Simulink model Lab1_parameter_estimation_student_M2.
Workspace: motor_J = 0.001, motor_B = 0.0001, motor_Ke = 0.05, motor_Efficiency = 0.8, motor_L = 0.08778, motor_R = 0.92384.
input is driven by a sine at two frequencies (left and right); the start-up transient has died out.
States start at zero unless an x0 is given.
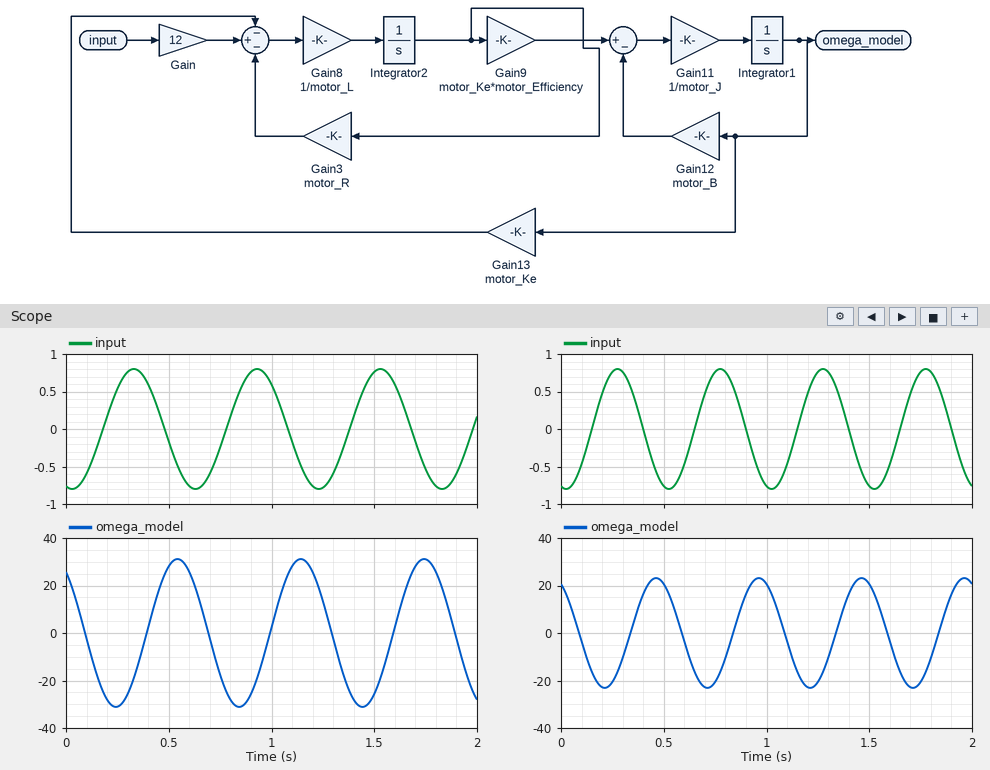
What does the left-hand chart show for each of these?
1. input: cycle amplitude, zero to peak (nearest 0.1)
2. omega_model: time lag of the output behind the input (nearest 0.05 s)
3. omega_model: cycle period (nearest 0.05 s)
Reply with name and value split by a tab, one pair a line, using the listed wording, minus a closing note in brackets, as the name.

input: cycle amplitude, zero to peak	0.8
omega_model: time lag of the output behind the input	0.20 s
omega_model: cycle period	0.60 s
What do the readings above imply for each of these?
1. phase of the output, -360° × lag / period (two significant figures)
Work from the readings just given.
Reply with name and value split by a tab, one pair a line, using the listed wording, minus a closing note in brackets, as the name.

phase of the output, -360° × lag / period	-120°
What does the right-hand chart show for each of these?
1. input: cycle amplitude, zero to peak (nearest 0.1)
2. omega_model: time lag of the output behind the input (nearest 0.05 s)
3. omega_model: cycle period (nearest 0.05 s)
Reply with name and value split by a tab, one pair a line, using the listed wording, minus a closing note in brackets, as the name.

input: cycle amplitude, zero to peak	0.8
omega_model: time lag of the output behind the input	0.20 s
omega_model: cycle period	0.50 s
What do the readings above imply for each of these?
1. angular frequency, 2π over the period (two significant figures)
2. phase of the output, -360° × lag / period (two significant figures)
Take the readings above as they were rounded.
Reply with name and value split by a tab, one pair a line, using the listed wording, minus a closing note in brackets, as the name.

angular frequency, 2π over the period	13 rad/s
phase of the output, -360° × lag / period	-140°
